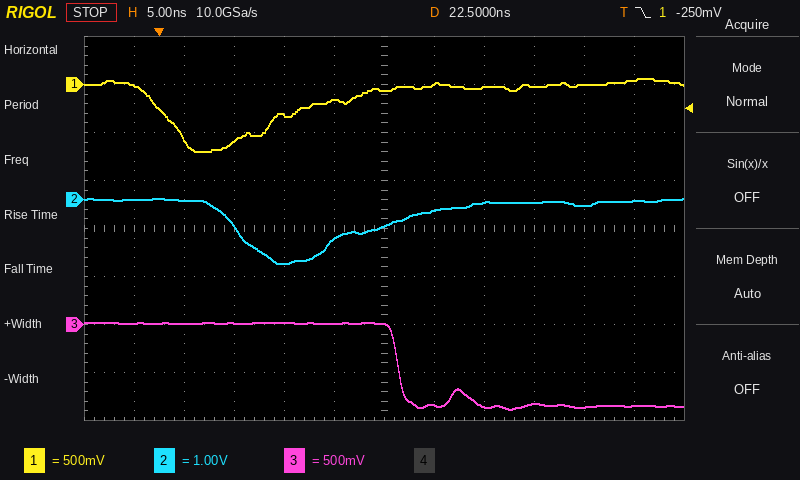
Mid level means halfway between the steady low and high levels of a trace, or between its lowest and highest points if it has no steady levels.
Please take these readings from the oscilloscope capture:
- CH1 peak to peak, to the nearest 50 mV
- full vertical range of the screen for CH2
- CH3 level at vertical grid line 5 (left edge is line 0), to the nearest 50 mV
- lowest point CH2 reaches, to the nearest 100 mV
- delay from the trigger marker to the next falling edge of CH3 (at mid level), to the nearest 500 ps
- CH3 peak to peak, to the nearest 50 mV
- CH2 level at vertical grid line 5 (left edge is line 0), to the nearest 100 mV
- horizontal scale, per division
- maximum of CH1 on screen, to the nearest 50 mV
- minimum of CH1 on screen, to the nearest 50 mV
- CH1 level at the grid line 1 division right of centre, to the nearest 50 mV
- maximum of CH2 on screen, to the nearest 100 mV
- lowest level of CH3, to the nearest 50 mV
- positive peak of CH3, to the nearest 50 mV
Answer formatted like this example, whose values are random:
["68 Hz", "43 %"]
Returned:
["750 mV", "8 V", "0 mV", "-1.3 V", "24.0 ns", "900 mV", "-800 mV", "5 ns", "50 mV", "-700 mV", "0 mV", "0.0 V", "-900 mV", "0 mV"]
